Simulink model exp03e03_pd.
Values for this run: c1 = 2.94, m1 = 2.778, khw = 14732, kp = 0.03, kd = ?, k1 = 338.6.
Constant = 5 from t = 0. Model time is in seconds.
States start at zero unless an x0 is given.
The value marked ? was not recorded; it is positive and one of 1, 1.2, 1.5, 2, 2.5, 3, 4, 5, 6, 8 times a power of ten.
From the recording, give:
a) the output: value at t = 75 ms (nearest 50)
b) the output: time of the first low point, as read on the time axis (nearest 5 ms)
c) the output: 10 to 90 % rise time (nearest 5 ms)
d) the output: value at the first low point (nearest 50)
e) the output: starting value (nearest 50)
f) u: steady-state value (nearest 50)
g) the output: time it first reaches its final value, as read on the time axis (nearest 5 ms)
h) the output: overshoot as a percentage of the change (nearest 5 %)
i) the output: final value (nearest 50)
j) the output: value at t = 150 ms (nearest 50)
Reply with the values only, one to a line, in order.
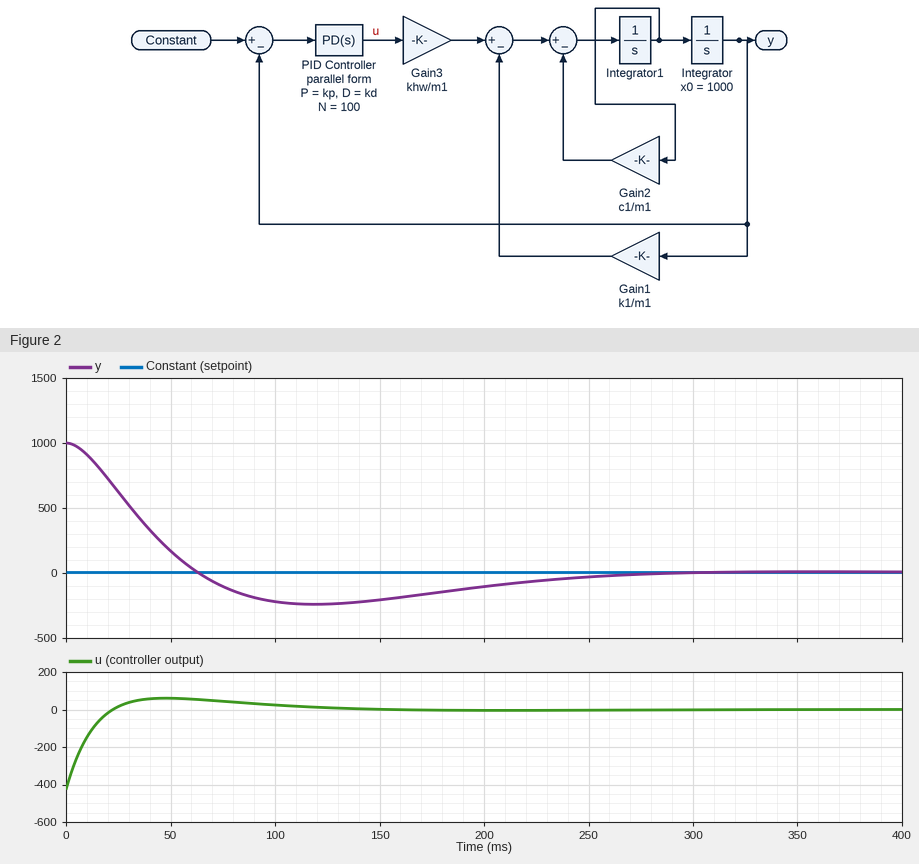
-100
120 ms
45 ms
-250
1000
0
65 ms
25 %
0
-200
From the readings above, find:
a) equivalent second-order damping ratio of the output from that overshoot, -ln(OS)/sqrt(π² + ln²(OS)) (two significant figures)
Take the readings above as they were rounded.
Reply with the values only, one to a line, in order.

0.40
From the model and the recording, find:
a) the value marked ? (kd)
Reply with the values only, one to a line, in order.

0.004
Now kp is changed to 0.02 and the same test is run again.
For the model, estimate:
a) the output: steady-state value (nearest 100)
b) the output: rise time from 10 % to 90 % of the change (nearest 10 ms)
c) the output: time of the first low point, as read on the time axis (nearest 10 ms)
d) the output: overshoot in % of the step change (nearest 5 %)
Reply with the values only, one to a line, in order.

0
50 ms
130 ms
20 %
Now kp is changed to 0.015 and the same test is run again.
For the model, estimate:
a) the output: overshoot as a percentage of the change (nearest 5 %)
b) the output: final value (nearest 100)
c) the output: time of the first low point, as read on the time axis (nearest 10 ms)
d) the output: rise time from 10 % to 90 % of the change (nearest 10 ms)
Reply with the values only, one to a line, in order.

20 %
0
130 ms
50 ms
